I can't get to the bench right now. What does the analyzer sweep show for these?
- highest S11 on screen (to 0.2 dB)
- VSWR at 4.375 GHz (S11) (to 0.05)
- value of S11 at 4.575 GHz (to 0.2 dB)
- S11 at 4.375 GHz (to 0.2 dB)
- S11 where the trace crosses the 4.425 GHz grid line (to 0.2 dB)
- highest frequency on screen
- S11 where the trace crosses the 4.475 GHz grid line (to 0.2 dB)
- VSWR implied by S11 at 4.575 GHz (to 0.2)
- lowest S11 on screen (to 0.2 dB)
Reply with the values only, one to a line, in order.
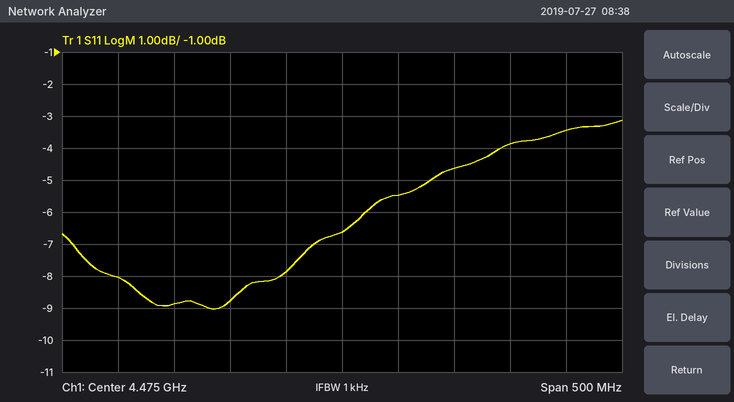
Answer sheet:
-3.2 dB
2.15
-4.6 dB
-8.8 dB
-7.8 dB
4.725 GHz
-6.6 dB
3.8
-9.0 dB
